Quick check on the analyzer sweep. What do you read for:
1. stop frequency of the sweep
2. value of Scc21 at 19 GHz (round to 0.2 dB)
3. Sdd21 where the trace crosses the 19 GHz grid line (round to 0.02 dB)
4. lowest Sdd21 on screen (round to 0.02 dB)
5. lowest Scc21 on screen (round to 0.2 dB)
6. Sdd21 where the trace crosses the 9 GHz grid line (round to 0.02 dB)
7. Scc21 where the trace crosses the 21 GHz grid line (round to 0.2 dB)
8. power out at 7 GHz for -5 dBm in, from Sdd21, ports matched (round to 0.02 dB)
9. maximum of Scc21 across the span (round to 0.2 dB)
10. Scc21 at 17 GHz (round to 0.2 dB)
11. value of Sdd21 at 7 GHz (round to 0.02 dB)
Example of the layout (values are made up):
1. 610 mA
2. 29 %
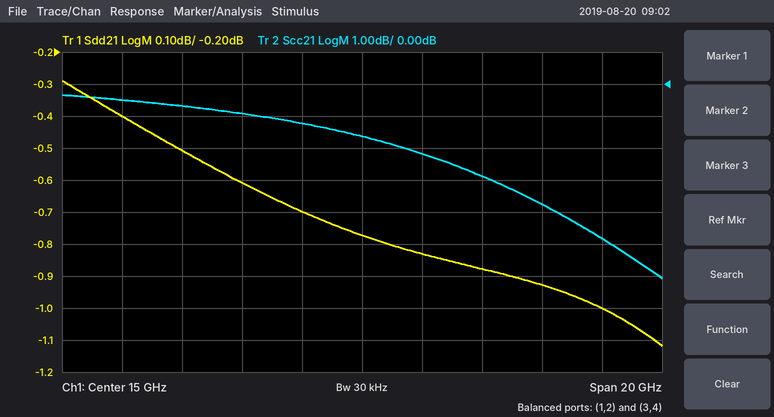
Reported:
1. 25 GHz
2. -2.8 dB
3. -0.88 dB
4. -1.12 dB
5. -6.0 dB
6. -0.50 dB
7. -3.8 dB
8. -5.40 dBm
9. -0.4 dB
10. -2.2 dB
11. -0.40 dB
